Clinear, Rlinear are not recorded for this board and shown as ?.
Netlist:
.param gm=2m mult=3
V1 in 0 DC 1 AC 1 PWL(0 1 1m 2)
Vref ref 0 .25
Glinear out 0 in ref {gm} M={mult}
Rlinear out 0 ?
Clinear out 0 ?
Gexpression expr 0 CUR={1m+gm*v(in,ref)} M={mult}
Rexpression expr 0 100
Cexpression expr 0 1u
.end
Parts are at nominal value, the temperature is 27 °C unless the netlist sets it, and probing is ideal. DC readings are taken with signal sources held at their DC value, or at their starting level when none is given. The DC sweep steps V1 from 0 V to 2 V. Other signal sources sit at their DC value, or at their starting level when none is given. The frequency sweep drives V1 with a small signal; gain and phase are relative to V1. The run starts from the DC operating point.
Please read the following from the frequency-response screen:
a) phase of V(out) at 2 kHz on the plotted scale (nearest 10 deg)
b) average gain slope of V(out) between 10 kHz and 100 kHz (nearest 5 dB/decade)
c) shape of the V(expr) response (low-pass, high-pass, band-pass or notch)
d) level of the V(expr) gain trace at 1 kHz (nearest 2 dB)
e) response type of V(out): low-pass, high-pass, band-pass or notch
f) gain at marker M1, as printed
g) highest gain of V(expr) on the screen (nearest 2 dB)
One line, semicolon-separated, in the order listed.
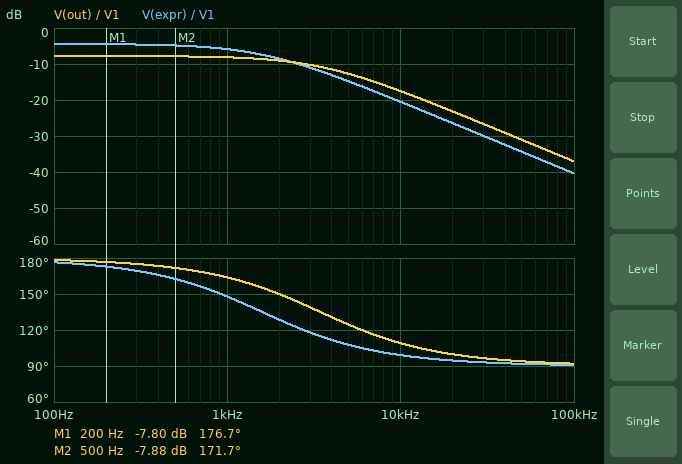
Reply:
150 deg; -20 dB/decade; low-pass; -6 dB; low-pass; -7.80 dB; -4 dB
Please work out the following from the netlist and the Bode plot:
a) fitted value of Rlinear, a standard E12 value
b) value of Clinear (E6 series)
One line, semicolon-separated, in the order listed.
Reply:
68 Ω; 680 nF
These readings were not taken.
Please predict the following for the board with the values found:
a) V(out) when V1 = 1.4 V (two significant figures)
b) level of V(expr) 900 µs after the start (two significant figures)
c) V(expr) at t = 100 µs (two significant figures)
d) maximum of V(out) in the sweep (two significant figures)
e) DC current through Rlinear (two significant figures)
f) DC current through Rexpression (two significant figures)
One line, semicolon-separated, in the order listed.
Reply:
-470 mV; -1.2 V; -770 mV; 100 mV; 4.5 mA; 7.5 mA
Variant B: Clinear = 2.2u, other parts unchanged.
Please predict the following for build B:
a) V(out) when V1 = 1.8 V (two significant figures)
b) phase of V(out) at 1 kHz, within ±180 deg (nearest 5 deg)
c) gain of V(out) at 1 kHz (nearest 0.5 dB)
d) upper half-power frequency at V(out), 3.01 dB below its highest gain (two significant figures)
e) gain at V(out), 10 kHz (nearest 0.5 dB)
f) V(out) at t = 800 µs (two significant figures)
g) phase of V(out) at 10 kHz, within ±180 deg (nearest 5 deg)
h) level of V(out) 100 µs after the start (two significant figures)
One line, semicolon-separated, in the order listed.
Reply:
-630 mV; 135 deg; -10.5 dB; 1.1 kHz; -27.5 dB; -570 mV; 95 deg; -320 mV
